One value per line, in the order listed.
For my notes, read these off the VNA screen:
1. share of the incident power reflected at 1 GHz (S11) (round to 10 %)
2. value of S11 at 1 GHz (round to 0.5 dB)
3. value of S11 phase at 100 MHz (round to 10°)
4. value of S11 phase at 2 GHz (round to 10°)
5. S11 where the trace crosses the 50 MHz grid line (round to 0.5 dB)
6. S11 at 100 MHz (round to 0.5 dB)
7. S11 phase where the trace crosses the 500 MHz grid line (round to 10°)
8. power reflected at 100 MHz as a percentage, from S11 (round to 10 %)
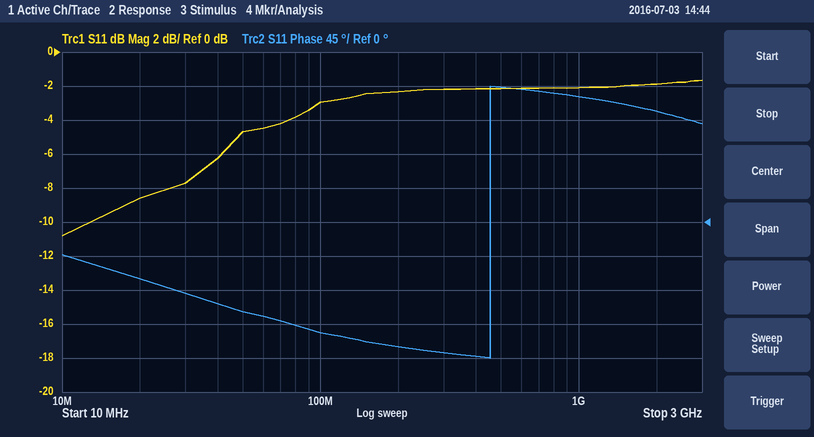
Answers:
60 %
-2.0 dB
-150°
150°
-4.5 dB
-3.0 dB
180°
50 %
